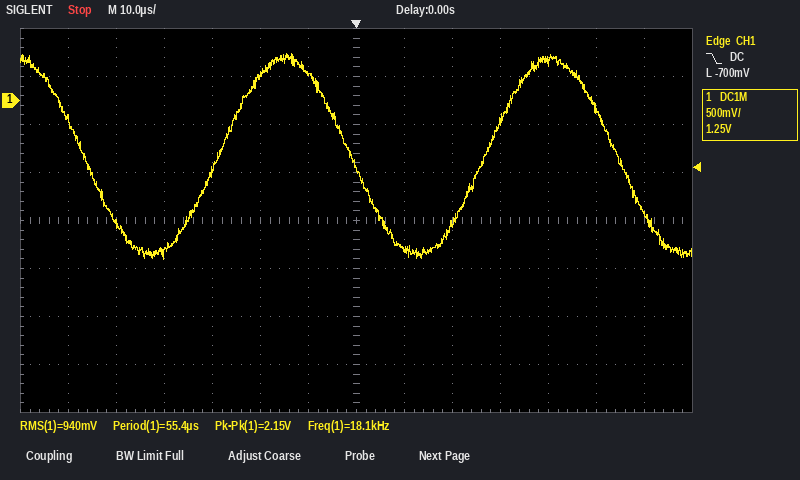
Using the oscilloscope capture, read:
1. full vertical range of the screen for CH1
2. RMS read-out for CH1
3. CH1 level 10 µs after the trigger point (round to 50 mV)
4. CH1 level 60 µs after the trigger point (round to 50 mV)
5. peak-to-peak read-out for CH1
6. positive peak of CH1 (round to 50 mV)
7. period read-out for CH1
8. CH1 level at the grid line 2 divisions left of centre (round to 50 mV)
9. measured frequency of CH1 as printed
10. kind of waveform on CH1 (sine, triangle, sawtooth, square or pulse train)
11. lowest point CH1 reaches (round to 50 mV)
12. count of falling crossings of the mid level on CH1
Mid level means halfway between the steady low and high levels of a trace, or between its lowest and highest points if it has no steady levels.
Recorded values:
4 V
940 mV
-1.55 V
-1.20 V
2.15 V
500 mV
55.4 µs
250 mV
18.1 kHz
sine
-1.65 V
3
